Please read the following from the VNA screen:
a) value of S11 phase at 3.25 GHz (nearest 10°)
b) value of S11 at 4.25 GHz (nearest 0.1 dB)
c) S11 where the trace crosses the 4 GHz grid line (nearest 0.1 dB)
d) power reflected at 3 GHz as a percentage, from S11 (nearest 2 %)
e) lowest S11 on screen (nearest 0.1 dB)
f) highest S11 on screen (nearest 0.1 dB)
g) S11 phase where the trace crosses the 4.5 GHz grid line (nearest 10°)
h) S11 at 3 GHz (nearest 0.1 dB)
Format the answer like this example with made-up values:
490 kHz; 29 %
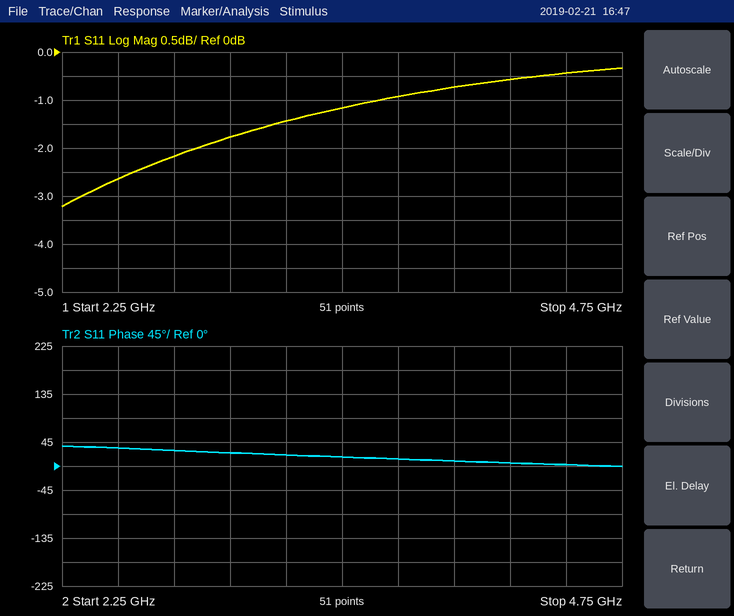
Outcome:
20°; -0.6 dB; -0.7 dB; 66 %; -3.2 dB; -0.3 dB; 0°; -1.8 dB
